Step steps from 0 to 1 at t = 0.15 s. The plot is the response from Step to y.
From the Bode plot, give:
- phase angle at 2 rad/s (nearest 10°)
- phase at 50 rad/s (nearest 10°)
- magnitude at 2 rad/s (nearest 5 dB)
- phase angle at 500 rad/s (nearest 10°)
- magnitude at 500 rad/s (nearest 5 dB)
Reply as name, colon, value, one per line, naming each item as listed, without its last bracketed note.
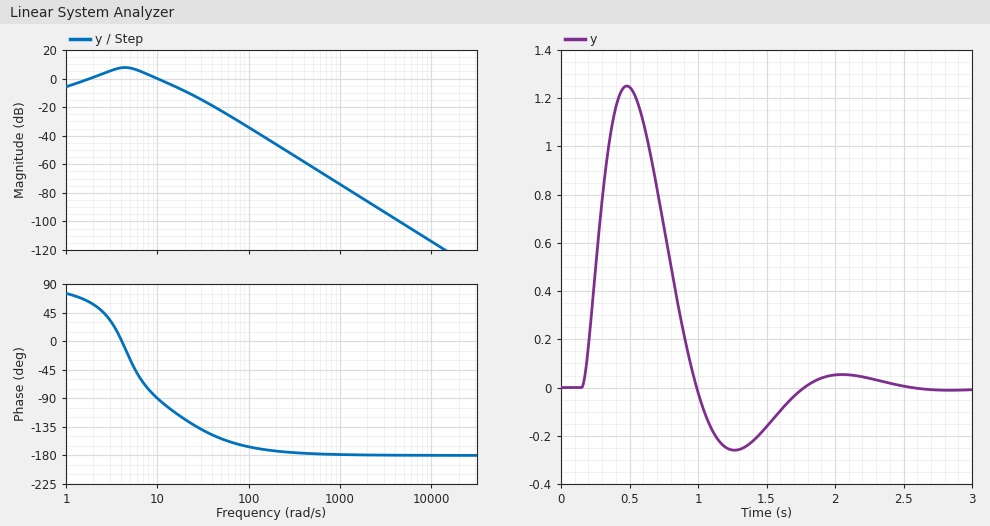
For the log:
phase angle at 2 rad/s: 60°
phase at 50 rad/s: -150°
magnitude at 2 rad/s: 0 dB
phase angle at 500 rad/s: -180°
magnitude at 500 rad/s: -60 dB
